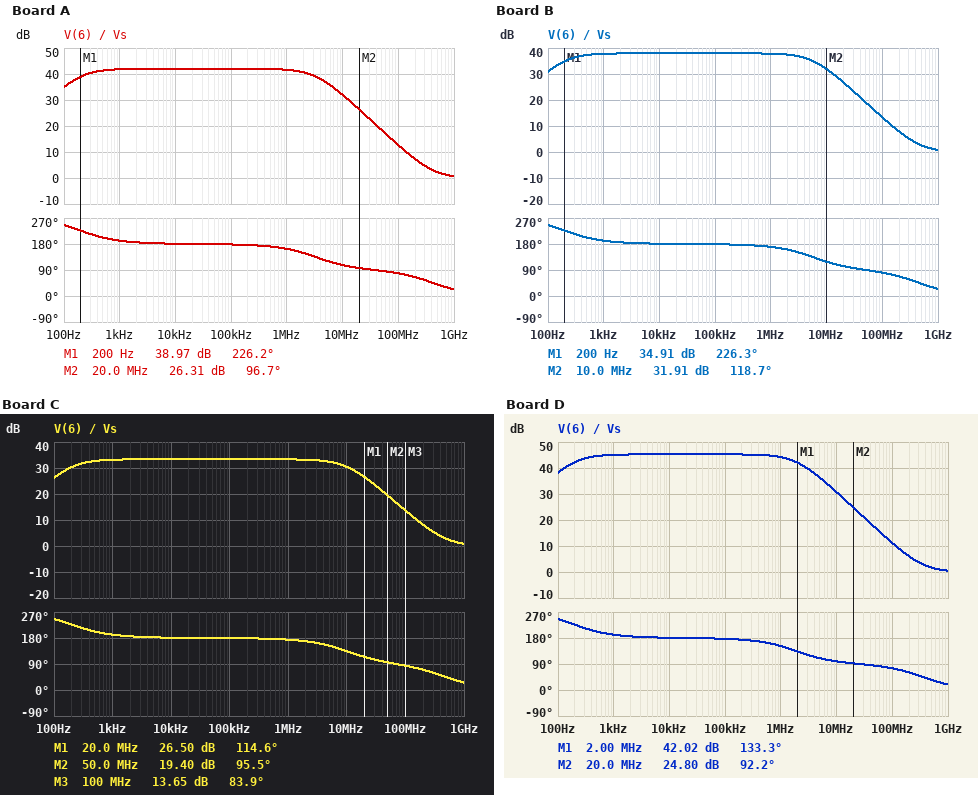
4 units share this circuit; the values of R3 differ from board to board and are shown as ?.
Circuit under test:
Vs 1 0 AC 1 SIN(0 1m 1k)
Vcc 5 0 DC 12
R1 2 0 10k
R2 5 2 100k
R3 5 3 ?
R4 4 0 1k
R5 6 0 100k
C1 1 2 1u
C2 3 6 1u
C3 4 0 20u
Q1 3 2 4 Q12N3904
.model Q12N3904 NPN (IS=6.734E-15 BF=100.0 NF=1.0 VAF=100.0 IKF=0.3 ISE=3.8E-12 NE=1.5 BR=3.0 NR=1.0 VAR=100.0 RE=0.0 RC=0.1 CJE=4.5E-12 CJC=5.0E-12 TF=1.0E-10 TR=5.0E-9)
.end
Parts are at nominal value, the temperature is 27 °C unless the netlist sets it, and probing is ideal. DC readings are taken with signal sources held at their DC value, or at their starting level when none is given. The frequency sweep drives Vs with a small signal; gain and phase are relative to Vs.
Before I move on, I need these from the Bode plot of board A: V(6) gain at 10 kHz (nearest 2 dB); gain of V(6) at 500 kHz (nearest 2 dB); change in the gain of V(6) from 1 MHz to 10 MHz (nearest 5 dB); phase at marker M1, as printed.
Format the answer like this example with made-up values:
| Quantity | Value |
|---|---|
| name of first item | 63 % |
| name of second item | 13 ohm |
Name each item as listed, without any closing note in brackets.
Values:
| Quantity | Value |
|---|---|
| V(6) gain at 10 kHz | 42 dB |
| gain of V(6) at 500 kHz | 42 dB |
| change in the gain of V(6) from 1 MHz to 10 MHz | -10 dB |
| phase at marker M1, as printed | 226.2 deg |
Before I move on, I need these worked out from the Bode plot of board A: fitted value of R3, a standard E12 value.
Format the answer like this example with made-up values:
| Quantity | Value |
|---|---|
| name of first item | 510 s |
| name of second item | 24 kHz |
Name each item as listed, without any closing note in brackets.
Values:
| Quantity | Value |
|---|---|
| fitted value of R3, a standard E12 value | 27 kΩ |
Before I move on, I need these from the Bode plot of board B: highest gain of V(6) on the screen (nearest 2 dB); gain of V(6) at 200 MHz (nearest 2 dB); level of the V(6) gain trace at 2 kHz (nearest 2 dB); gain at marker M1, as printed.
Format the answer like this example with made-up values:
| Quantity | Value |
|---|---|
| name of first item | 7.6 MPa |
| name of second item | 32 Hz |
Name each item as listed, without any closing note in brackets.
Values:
| Quantity | Value |
|---|---|
| highest gain of V(6) on the screen | 38 dB |
| gain of V(6) at 200 MHz | 8 dB |
| level of the V(6) gain trace at 2 kHz | 38 dB |
| gain at marker M1, as printed | 34.91 dB |
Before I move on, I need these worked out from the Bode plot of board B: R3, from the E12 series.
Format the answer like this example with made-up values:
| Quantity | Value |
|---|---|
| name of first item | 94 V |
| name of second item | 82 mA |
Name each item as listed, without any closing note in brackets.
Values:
| Quantity | Value |
|---|---|
| R3, from the E12 series | 15 kΩ |
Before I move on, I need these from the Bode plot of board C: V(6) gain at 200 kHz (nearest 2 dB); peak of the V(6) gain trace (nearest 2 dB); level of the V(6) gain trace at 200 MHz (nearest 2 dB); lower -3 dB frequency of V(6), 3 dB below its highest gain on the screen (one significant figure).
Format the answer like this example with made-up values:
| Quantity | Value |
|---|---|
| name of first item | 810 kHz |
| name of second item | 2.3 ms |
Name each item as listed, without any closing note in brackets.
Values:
| Quantity | Value |
|---|---|
| V(6) gain at 200 kHz | 34 dB |
| peak of the V(6) gain trace | 34 dB |
| level of the V(6) gain trace at 200 MHz | 8 dB |
| lower -3 dB frequency of V(6), 3 dB below its highest gain on the screen | 200 Hz |
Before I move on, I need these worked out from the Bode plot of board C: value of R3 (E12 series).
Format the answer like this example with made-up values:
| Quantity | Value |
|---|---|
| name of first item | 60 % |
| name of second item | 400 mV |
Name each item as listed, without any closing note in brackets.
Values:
| Quantity | Value |
|---|---|
| value of R3 | 8.2 kΩ |
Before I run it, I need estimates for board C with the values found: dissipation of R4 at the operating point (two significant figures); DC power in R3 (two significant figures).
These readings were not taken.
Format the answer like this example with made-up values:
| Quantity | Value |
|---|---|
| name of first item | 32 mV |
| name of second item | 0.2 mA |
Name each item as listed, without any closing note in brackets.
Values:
| Quantity | Value |
|---|---|
| dissipation of R4 at the operating point | 37 µW |
| DC power in R3 | 210 µW |
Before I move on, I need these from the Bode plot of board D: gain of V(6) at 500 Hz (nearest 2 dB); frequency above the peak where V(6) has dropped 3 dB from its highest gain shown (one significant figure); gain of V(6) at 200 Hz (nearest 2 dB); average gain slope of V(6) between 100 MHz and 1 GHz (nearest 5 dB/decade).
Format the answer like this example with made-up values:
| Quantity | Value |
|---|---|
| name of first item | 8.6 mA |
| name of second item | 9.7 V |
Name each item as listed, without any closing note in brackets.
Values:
| Quantity | Value |
|---|---|
| gain of V(6) at 500 Hz | 44 dB |
| frequency above the peak where V(6) has dropped 3 dB from its highest gain shown | 2 MHz |
| gain of V(6) at 200 Hz | 42 dB |
| average gain slope of V(6) between 100 MHz and 1 GHz | -10 dB/decade |
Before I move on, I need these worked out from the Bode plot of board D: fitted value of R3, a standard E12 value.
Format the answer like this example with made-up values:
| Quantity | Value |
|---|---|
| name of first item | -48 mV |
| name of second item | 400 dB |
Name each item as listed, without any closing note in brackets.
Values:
| Quantity | Value |
|---|---|
| fitted value of R3, a standard E12 value | 47 kΩ |
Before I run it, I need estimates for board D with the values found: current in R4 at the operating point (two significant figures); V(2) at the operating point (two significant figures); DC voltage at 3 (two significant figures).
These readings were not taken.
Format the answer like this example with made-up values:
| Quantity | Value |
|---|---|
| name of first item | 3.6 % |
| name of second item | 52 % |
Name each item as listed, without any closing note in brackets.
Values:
| Quantity | Value |
|---|---|
| current in R4 at the operating point | 190 µA |
| V(2) at the operating point | 800 mV |
| DC voltage at 3 | 4.7 V |
